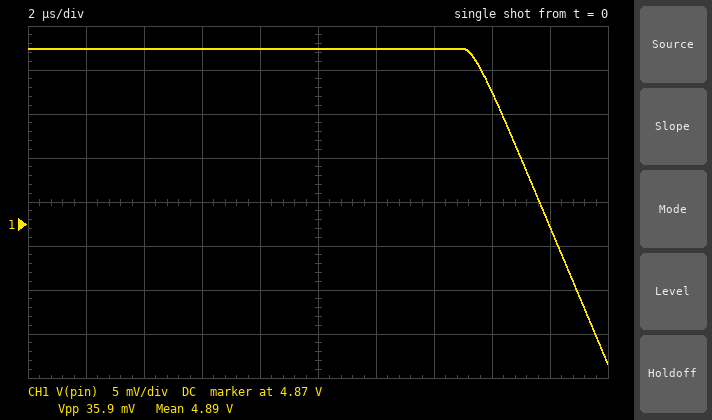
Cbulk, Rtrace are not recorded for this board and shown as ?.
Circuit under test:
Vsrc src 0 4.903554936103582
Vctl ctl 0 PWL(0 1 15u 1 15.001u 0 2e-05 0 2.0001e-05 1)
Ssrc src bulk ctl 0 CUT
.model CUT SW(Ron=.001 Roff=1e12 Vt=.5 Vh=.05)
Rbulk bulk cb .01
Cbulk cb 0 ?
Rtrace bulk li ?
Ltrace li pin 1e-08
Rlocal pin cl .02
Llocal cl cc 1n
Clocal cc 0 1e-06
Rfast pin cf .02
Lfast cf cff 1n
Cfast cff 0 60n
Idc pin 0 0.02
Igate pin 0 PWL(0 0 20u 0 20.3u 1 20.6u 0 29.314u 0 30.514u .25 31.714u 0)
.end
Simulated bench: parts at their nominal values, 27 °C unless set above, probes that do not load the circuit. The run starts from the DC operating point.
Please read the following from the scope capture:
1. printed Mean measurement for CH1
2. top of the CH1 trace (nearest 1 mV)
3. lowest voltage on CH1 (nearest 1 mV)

4.89 V
4.890 V
4.854 V
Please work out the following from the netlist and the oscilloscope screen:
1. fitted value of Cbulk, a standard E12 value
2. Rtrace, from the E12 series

1.5 µF
0.68 Ω
